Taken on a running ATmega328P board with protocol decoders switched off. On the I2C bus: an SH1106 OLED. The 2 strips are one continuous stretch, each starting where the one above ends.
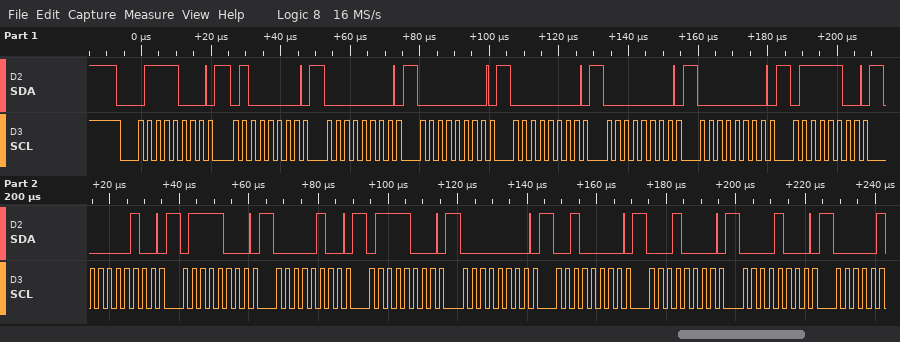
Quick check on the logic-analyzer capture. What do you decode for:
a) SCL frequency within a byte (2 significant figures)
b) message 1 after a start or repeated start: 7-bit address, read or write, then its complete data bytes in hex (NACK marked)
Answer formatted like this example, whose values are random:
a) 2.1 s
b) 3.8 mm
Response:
a) 400 kHz
b) 0x3C write: 40 00 00 00 00 00 7C 04 78 04 78 00 20 10 08
